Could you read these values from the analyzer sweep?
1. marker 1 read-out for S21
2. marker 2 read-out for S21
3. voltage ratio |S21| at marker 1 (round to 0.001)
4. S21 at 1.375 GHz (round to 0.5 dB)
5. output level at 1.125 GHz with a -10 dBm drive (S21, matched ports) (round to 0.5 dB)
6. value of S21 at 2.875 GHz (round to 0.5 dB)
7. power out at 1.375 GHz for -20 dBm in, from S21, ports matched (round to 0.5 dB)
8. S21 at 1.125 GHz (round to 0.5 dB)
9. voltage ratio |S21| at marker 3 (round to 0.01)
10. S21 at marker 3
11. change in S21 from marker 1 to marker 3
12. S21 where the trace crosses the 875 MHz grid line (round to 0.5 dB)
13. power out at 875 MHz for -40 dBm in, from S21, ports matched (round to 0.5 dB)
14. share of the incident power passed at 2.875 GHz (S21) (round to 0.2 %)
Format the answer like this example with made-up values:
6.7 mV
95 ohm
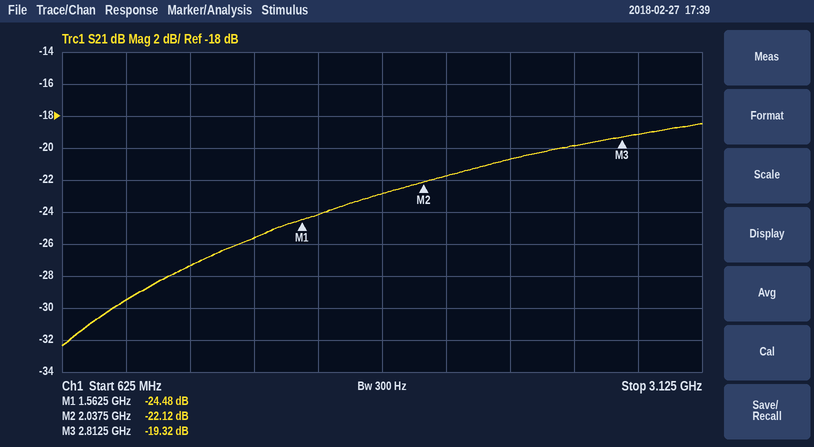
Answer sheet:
-24.48 dB
-22.12 dB
0.060
-25.5 dB
-37.5 dBm
-19.0 dB
-45.5 dBm
-27.5 dB
0.11
-19.32 dB
5.16 dB
-29.5 dB
-69.5 dBm
1.2 %
